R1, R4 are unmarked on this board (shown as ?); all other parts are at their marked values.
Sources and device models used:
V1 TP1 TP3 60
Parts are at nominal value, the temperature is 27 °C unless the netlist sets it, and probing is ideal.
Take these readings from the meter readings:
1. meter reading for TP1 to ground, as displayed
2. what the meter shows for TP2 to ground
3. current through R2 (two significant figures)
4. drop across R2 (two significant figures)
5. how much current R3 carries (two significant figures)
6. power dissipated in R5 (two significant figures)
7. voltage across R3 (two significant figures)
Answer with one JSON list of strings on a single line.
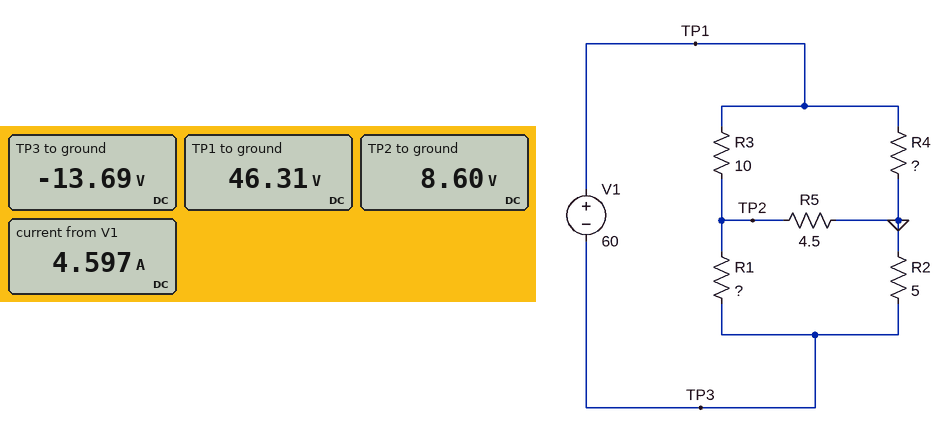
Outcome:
["46.31 V", "8.60 V", "2.7 A", "14 V", "3.8 A", "16 W", "38 V"]
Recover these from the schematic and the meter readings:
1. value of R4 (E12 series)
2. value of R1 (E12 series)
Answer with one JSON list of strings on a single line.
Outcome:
["56 Ω", "12 Ω"]
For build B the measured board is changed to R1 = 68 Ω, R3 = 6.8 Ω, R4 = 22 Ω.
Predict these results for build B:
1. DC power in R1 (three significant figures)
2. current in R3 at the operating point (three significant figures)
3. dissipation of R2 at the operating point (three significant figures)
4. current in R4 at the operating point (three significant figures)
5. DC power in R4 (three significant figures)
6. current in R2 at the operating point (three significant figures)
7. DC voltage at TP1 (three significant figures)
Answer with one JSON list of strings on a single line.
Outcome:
["19.4 W", "3.48 A", "107 W", "1.68 A", "61.9 W", "4.62 A", "36.9 V"]
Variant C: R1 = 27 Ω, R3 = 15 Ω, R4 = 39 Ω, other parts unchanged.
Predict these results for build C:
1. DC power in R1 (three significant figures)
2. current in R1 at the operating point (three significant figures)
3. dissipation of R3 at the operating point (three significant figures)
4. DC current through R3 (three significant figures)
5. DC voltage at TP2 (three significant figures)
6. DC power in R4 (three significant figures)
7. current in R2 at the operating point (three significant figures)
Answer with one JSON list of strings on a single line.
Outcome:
["18.1 W", "818 mA", "95.8 W", "2.53 A", "7.69 V", "53.3 W", "2.88 A"]
